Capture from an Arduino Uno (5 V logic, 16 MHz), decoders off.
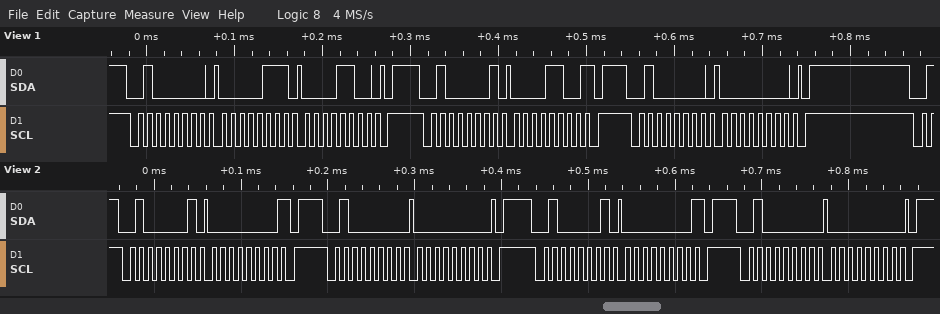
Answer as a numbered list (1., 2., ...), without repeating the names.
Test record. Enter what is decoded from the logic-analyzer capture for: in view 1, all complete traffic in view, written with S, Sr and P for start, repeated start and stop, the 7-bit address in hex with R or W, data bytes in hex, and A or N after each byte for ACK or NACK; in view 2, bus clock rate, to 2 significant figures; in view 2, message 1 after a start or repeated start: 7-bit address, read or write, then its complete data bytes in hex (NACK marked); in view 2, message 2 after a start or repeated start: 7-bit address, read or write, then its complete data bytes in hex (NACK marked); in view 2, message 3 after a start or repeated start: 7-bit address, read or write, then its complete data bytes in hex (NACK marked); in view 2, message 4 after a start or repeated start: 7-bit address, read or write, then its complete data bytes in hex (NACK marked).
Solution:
1. S 20W A 07 A 0C A P S 20R A 0C N P S 20W A 00 A P
2. 100 kHz
3. 0x20 read: 00 NACK
4. 0x20 write: 00
5. 0x20 read: 00 NACK
6. 0x20 write: 00
